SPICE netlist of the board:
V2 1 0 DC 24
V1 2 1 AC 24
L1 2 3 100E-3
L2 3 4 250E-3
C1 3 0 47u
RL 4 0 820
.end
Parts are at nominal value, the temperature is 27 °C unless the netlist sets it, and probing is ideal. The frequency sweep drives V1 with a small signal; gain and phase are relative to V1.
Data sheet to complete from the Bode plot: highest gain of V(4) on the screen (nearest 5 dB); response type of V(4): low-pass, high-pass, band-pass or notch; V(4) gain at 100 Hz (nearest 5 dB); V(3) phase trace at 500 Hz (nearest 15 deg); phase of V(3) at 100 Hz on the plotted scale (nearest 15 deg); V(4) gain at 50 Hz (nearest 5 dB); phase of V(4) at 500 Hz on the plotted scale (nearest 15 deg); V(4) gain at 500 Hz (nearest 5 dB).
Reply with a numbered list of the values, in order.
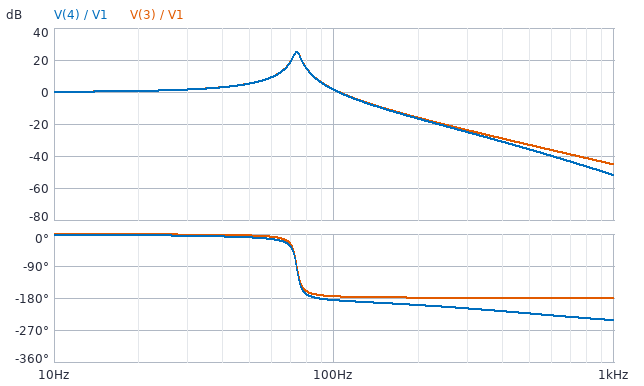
1. 25 dB
2. low-pass
3. 0 dB
4. -180 deg
5. -180 deg
6. 5 dB
7. -225 deg
8. -35 dB
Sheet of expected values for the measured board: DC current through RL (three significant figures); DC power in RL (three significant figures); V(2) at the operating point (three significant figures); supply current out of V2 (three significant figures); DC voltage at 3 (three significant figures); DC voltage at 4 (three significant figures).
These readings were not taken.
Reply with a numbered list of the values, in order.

1. 29.3 mA
2. 702 mW
3. 24.0 V
4. 29.3 mA
5. 24.0 V
6. 24.0 V
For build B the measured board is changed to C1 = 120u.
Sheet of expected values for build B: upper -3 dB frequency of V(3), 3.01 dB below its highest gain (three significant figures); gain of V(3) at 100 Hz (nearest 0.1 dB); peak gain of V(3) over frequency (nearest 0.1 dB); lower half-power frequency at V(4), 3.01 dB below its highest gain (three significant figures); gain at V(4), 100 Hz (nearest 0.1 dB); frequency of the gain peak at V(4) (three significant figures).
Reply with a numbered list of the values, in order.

1. 46.8 Hz
2. -11.4 dB
3. 29.1 dB
4. 45.2 Hz
5. -11.6 dB
6. 46.0 Hz
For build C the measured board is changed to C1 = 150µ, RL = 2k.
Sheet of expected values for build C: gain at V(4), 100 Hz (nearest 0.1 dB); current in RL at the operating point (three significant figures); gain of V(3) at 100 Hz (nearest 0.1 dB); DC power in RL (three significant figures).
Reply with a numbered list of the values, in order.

1. -13.9 dB
2. 12.0 mA
3. -13.8 dB
4. 288 mW
